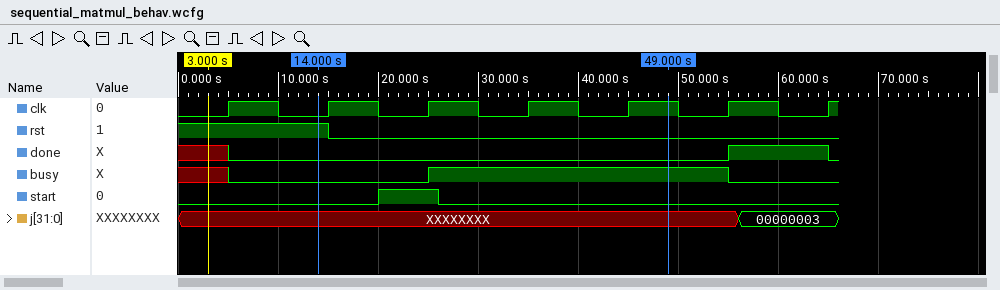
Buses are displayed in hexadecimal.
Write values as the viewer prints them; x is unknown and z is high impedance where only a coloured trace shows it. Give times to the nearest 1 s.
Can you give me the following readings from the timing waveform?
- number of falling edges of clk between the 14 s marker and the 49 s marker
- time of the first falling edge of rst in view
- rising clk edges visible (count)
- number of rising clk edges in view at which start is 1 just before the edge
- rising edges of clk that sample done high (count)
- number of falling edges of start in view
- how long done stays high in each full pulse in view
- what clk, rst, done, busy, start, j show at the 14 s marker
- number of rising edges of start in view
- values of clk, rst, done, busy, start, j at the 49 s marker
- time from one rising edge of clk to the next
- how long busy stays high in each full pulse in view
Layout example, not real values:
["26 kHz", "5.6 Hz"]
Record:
["3", "15 s", "7", "1", "1", "1", "10 s", "clk=0, rst=1, done=0, busy=0, start=0, j=XXXXXXXX", "1", "clk=1, rst=0, done=0, busy=1, start=0, j=XXXXXXXX", "10 s", "30 s"]
